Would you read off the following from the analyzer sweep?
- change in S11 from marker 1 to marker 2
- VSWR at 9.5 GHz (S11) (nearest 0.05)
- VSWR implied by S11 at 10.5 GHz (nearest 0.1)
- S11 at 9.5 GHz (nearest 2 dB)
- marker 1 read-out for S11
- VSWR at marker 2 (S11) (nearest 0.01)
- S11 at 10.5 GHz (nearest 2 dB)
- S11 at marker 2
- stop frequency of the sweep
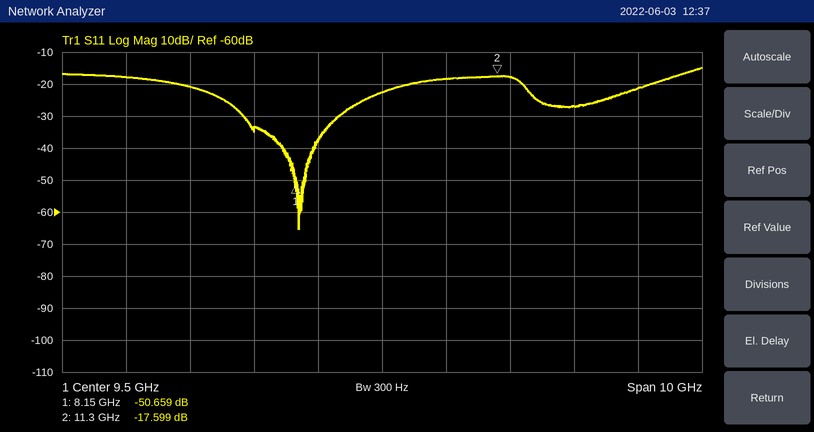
33.060 dB
1.15
1.3
-22 dB
-50.659 dB
1.30
-18 dB
-17.599 dB
14.5 GHz
